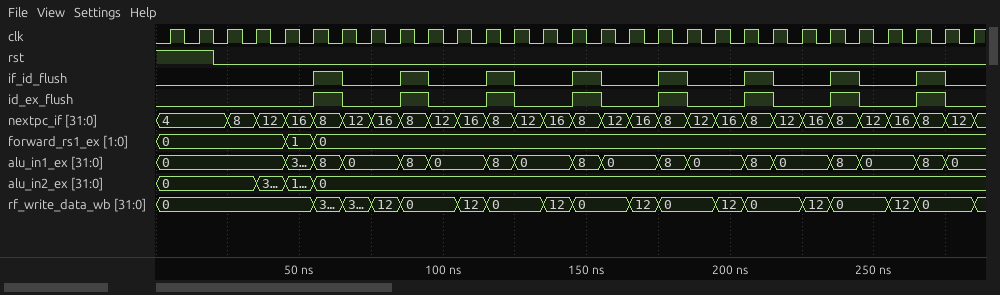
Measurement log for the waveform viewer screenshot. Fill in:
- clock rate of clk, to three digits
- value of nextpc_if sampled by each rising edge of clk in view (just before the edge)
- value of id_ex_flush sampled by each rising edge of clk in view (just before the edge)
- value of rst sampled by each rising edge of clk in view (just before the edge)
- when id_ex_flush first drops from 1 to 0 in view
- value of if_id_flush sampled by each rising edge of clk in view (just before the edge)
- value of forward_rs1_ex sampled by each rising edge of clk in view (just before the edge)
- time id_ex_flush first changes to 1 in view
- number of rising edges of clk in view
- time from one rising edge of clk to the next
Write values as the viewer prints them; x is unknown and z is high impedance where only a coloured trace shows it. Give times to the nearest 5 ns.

100 MHz
4, 4, 4, 8, 12, 16, 8, 12, 16, 8, 12, 16, 8, 12, 16, 8, 12, 16, 8, 12, 16, 8, 12, 16, 8, 12, 16, 8, 12
0 0 0 0 0 0 1 0 0 1 0 0 1 0 0 1 0 0 1 0 0 1 0 0 1 0 0 1 0
1 1 0 0 0 0 0 0 0 0 0 0 0 0 0 0 0 0 0 0 0 0 0 0 0 0 0 0 0
65 ns
0 0 0 0 0 0 1 0 0 1 0 0 1 0 0 1 0 0 1 0 0 1 0 0 1 0 0 1 0
0, 0, 0, 0, 0, 1, 0, 0, 0, 0, 0, 0, 0, 0, 0, 0, 0, 0, 0, 0, 0, 0, 0, 0, 0, 0, 0, 0, 0
55 ns
29
10 ns
